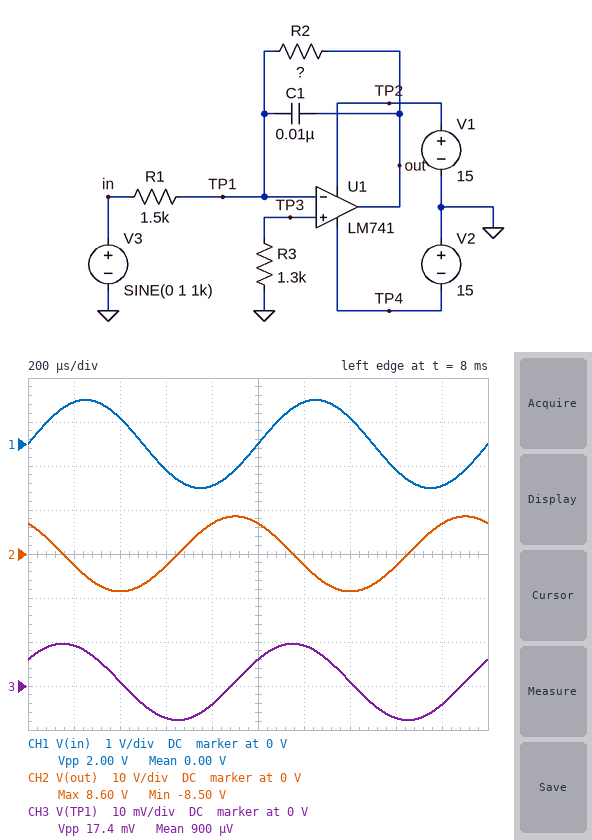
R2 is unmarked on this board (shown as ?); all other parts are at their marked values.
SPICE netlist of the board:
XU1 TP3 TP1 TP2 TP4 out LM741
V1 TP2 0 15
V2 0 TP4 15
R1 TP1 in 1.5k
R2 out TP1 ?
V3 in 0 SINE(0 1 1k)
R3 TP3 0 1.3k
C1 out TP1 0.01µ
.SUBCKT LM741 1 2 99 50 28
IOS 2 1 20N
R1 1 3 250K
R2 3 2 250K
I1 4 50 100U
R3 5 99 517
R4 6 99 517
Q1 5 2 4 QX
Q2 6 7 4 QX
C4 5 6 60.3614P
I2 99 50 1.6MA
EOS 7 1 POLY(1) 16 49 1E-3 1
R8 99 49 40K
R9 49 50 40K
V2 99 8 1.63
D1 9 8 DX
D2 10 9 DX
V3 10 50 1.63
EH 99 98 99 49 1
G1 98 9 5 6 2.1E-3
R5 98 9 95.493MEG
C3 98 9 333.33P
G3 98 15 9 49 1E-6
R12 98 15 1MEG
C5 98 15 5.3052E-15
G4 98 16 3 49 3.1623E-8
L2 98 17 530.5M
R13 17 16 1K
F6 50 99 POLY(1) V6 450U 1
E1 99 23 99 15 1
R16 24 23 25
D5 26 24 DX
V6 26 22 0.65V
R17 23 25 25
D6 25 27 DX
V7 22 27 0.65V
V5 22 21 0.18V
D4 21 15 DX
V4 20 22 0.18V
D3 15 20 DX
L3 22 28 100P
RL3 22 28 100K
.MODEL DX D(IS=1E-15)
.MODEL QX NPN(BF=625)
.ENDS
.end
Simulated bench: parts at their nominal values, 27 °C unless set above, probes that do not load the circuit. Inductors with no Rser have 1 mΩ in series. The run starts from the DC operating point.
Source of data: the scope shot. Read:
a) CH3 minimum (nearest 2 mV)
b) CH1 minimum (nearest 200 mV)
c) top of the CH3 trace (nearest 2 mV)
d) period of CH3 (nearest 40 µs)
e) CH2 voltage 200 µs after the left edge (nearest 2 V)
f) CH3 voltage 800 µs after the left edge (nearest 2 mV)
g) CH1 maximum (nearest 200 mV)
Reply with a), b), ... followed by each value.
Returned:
a) -8 mV
b) -1.0 V
c) 10 mV
d) 1.00 ms
e) -2 V
f) -4 mV
g) 1.0 V
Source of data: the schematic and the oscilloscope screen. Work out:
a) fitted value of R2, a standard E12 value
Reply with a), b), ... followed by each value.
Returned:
a) 22 kΩ
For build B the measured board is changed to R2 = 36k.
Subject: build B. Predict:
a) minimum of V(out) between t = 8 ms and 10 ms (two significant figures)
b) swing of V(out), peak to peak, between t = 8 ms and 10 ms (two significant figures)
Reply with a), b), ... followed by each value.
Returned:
a) -9.6 V
b) 19 V
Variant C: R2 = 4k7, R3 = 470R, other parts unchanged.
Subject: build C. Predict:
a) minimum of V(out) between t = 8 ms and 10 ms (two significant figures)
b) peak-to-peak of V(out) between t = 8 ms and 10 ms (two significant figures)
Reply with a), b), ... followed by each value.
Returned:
a) -3.0 V
b) 6.0 V
